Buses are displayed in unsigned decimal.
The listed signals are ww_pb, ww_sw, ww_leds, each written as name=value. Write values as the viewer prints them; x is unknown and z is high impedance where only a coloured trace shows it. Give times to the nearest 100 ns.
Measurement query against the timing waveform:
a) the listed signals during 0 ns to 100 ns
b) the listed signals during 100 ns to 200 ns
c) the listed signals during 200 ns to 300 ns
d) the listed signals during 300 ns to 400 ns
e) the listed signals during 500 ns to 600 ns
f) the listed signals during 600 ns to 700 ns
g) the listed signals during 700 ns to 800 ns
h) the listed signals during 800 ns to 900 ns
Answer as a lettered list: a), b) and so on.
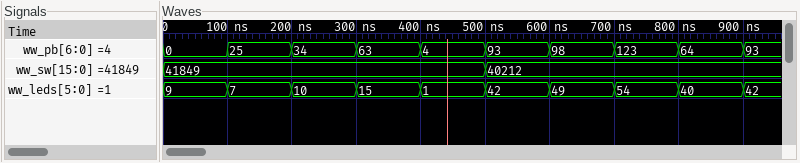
a) ww_pb=0, ww_sw=41849, ww_leds=9
b) ww_pb=25, ww_sw=41849, ww_leds=7
c) ww_pb=34, ww_sw=41849, ww_leds=10
d) ww_pb=63, ww_sw=41849, ww_leds=15
e) ww_pb=93, ww_sw=40212, ww_leds=42
f) ww_pb=98, ww_sw=40212, ww_leds=49
g) ww_pb=123, ww_sw=40212, ww_leds=54
h) ww_pb=64, ww_sw=40212, ww_leds=40
